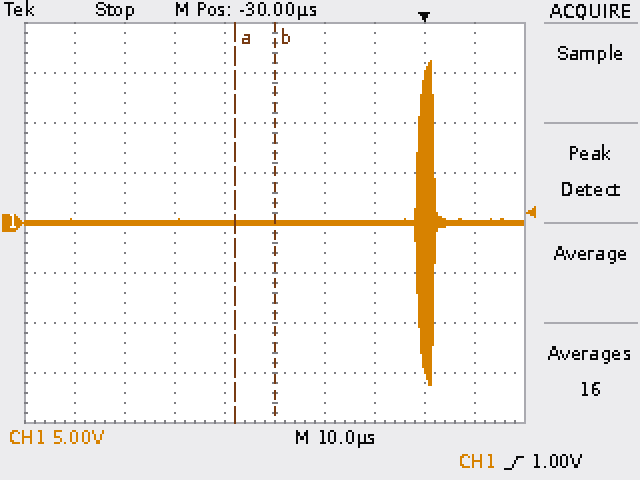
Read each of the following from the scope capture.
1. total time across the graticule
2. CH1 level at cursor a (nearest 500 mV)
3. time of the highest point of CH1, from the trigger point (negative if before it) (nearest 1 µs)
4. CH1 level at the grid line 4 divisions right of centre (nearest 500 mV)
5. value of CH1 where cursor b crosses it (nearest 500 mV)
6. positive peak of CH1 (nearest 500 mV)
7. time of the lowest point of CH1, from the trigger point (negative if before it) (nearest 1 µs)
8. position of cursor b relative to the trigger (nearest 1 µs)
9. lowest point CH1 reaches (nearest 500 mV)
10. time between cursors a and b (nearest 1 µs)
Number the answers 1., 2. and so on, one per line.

1. 100 µs
2. 0.0 V
3. +1 µs
4. 0.0 V
5. 0.0 V
6. 16.0 V
7. +1 µs
8. -30 µs
9. -16.0 V
10. 8 µs
